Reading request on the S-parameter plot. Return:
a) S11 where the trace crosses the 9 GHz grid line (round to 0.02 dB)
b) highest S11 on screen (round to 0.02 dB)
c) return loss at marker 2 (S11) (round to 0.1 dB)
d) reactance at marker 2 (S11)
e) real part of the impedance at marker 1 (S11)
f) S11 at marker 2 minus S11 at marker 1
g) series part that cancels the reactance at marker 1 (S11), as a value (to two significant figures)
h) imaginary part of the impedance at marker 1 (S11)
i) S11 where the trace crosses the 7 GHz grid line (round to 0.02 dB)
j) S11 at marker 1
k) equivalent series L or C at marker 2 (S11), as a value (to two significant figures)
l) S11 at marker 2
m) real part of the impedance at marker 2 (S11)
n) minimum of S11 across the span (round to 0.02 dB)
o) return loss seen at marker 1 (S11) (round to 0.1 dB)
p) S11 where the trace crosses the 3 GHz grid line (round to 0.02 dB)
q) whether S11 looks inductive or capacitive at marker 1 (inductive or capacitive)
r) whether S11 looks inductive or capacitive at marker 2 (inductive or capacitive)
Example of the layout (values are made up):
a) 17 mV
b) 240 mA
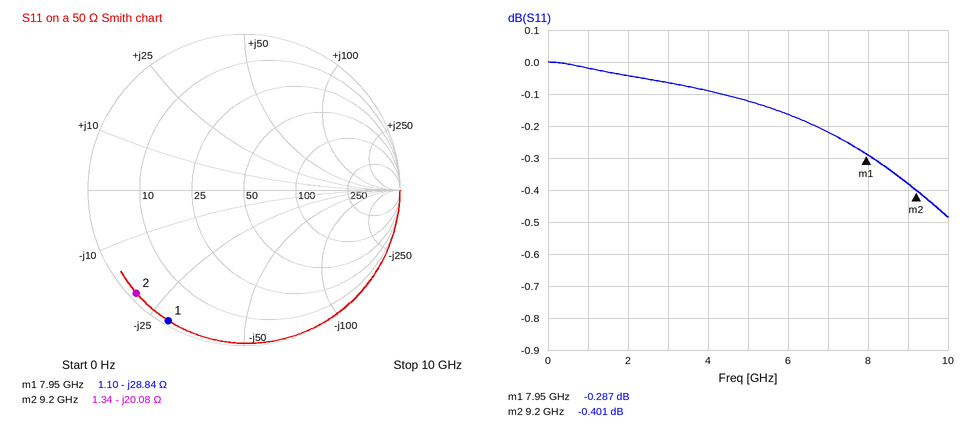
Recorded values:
a) -0.38 dB
b) 0.00 dB
c) 0.4 dB
d) -20.08 Ω
e) 1.10 Ω
f) -0.114 dB
g) 580 pH
h) -28.84 Ω
i) -0.22 dB
j) -0.287 dB
k) 860 fF
l) -0.401 dB
m) 1.34 Ω
n) -0.48 dB
o) 0.3 dB
p) -0.06 dB
q) capacitive
r) capacitive
